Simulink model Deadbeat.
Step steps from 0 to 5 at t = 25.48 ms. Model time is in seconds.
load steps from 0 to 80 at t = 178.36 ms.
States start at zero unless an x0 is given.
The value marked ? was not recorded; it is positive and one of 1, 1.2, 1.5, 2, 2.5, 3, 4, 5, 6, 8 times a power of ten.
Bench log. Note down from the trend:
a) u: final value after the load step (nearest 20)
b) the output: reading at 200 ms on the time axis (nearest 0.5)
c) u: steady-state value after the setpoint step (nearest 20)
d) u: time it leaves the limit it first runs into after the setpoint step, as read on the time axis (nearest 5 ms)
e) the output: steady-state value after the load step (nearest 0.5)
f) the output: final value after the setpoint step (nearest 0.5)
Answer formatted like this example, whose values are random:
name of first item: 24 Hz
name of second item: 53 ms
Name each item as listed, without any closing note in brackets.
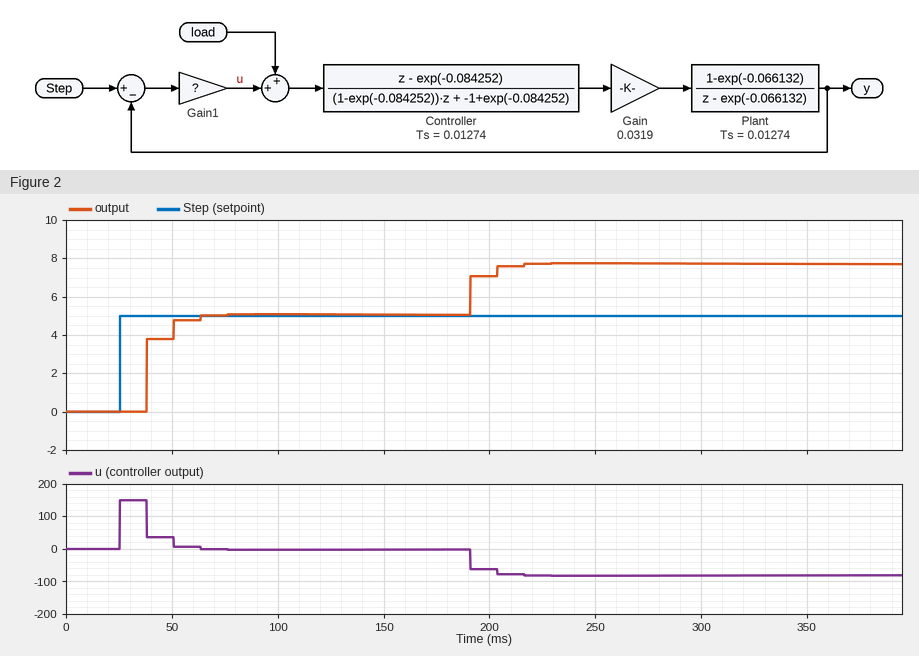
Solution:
u: final value after the load step: -80
the output: reading at 200 ms on the time axis: 7.0
u: steady-state value after the setpoint step: 0
u: time it leaves the limit it first runs into after the setpoint step, as read on the time axis: 40 ms
the output: steady-state value after the load step: 7.5
the output: final value after the setpoint step: 5.0
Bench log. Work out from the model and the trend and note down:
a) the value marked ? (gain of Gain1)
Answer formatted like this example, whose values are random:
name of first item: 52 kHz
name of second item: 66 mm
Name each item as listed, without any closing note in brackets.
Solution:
the value marked ?: 30
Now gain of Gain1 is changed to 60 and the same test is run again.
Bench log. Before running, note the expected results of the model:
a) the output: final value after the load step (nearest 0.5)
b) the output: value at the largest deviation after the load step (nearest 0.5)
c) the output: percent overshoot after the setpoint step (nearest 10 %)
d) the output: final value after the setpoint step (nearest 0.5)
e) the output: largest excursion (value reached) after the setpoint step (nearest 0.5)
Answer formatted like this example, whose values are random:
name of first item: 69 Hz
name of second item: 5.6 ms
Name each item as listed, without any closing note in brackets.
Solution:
the output: final value after the load step: 6.5
the output: value at the largest deviation after the load step: 7.0
the output: percent overshoot after the setpoint step: 50 %
the output: final value after the setpoint step: 5.0
the output: largest excursion (value reached) after the setpoint step: 7.5
